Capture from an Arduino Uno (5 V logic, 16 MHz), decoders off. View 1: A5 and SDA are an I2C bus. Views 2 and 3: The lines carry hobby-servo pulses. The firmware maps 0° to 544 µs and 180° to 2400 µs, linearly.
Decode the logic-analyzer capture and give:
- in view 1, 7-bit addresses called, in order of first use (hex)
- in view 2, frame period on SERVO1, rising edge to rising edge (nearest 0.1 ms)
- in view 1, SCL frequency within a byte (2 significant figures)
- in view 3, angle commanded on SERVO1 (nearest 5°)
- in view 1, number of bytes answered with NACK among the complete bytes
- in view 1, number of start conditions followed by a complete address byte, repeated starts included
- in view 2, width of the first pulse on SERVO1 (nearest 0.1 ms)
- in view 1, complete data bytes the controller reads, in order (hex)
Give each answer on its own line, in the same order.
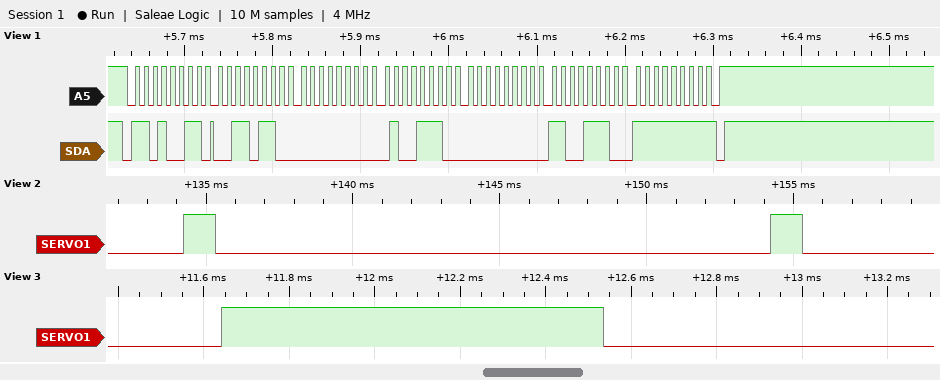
0x69
20.0 ms
100 kHz
35°
1
1
1.1 ms
36 00 4E 00 CE FF
